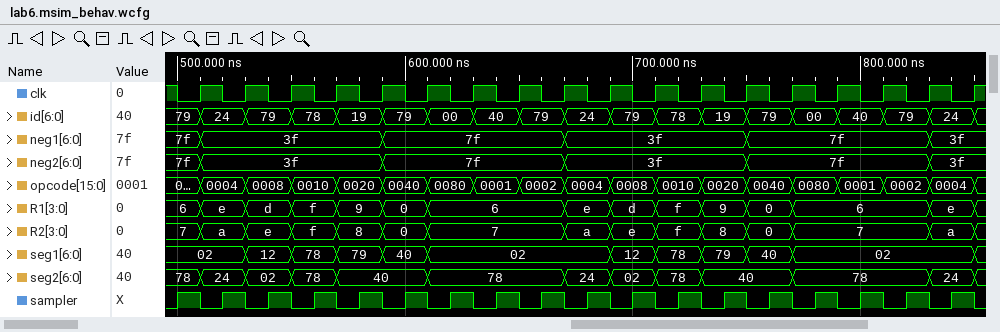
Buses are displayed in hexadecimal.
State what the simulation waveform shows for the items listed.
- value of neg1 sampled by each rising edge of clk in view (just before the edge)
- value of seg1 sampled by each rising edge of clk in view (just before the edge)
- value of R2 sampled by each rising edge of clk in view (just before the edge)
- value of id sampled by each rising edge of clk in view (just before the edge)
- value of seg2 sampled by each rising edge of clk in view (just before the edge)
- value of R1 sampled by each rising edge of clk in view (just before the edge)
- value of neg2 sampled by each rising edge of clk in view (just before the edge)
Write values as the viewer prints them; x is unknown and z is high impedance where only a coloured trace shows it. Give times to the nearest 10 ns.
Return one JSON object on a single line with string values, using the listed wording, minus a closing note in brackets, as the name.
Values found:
{"value of neg1 sampled by each rising edge of clk in view": "7f, 3f, 3f, 3f, 3f, 7f, 7f, 7f, 7f, 3f, 3f, 3f, 3f, 7f, 7f, 7f, 7f, 3f", "value of seg1 sampled by each rising edge of clk in view": "02, 02, 12, 78, 79, 40, 02, 02, 02, 02, 12, 78, 79, 40, 02, 02, 02, 02", "value of R2 sampled by each rising edge of clk in view": "7, a, e, f, 8, 0, 7, 7, 7, a, e, f, 8, 0, 7, 7, 7, a", "value of id sampled by each rising edge of clk in view": "79, 24, 79, 78, 19, 79, 00, 40, 79, 24, 79, 78, 19, 79, 00, 40, 79, 24", "value of seg2 sampled by each rising edge of clk in view": "78, 24, 02, 78, 40, 40, 78, 78, 78, 24, 02, 78, 40, 40, 78, 78, 78, 24", "value of R1 sampled by each rising edge of clk in view": "6, e, d, f, 9, 0, 6, 6, 6, e, d, f, 9, 0, 6, 6, 6, e", "value of neg2 sampled by each rising edge of clk in view": "7f, 3f, 3f, 3f, 3f, 7f, 7f, 7f, 7f, 3f, 3f, 3f, 3f, 7f, 7f, 7f, 7f, 3f"}
